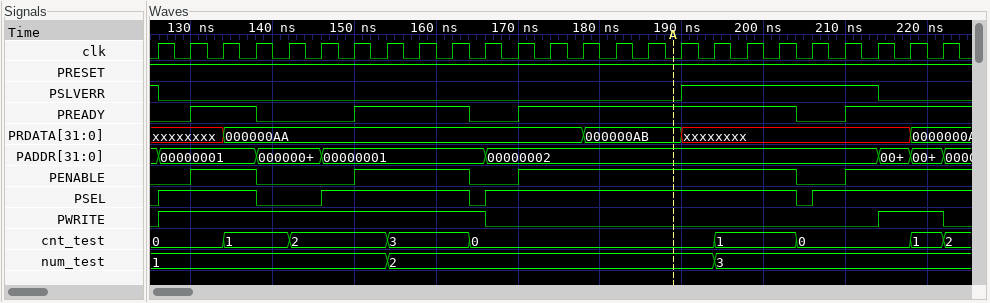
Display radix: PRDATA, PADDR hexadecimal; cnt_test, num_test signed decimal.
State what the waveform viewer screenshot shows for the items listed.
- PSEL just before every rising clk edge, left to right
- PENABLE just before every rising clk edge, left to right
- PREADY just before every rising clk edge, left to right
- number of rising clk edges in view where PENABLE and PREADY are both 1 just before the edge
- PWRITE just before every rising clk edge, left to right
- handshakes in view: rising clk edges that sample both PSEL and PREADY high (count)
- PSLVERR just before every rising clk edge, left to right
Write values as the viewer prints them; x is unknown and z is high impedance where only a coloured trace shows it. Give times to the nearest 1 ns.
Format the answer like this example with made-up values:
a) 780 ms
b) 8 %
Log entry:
a) 0 1 1 1 0 0 1 1 1 1 0 1 1 1 1 1 1 1 1 1 0 1 1 1 1
b) 0 0 1 1 0 0 0 1 1 1 0 0 1 1 1 1 1 1 1 1 0 0 1 1 1
c) 0 0 1 1 0 0 0 1 1 1 0 0 1 1 1 1 1 1 1 1 0 0 1 1 1
d) 16
e) 0 1 1 1 1 1 1 1 1 1 1 0 0 0 0 0 0 0 0 0 0 0 0 1 1
f) 16
g) 1 0 0 0 0 0 0 0 0 0 0 0 0 0 0 0 0 1 1 1 1 1 1 0 0
